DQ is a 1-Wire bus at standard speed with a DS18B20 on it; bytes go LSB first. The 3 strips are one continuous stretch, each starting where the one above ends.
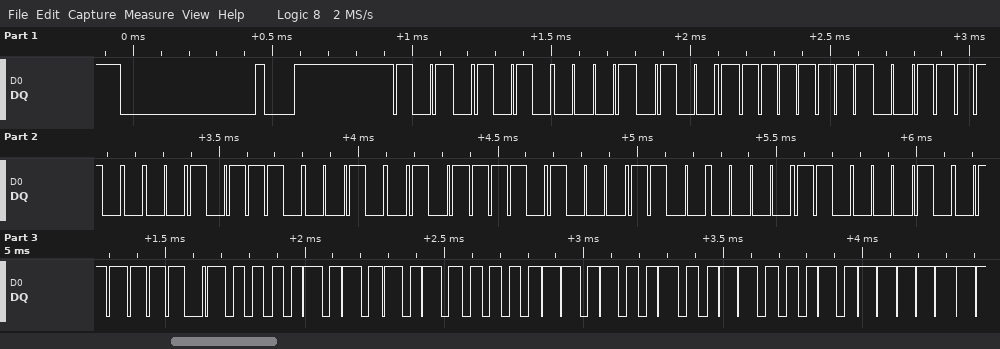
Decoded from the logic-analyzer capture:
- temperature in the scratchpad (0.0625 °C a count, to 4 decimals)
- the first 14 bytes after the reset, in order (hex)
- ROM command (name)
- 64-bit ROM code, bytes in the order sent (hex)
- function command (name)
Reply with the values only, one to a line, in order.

85.0000 °C
55 28 FF 3C 74 A4 17 03 43 BE 50 05 4B 46
Match ROM
28 FF 3C 74 A4 17 03 43
Read Scratchpad
